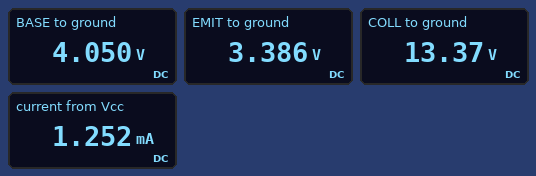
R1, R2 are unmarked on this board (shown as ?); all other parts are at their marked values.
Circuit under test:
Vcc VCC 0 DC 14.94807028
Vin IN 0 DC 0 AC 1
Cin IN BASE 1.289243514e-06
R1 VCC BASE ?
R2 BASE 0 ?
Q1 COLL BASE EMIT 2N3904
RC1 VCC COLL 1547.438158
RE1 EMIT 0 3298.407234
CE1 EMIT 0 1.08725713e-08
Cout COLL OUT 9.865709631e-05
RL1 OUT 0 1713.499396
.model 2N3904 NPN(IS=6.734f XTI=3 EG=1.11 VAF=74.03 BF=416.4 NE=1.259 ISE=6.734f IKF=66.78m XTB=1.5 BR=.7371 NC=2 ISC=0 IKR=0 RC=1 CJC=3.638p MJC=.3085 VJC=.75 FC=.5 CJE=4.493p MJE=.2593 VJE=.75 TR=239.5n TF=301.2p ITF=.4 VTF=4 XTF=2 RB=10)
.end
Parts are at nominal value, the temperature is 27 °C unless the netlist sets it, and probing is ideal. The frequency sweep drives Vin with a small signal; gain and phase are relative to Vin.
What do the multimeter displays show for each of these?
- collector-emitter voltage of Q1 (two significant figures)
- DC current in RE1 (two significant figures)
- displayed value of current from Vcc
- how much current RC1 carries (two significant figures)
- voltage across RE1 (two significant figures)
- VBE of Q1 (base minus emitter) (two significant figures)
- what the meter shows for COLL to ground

10 V
1.0 mA
1.252 mA
1.0 mA
3.4 V
660 mV
13.37 V
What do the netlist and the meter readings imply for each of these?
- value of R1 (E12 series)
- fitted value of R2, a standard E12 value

47 kΩ
18 kΩ
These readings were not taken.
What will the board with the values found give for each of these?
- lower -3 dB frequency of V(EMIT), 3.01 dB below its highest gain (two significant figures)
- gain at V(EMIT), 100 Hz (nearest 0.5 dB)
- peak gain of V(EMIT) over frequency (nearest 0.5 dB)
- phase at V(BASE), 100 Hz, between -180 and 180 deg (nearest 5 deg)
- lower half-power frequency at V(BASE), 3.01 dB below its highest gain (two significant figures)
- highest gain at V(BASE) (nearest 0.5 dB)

9.7 Hz
0 dB
0 dB
5 deg
9.7 Hz
0 dB
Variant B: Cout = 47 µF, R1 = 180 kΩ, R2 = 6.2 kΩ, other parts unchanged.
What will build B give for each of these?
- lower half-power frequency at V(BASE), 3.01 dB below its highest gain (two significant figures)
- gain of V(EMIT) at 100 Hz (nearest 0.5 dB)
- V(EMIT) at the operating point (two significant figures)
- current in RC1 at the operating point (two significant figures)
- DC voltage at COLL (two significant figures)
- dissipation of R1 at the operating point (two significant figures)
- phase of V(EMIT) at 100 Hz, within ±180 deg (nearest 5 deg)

21 Hz
-16.0 dB
5.0 mV
1.5 µA
15 V
1.2 mW
10 deg
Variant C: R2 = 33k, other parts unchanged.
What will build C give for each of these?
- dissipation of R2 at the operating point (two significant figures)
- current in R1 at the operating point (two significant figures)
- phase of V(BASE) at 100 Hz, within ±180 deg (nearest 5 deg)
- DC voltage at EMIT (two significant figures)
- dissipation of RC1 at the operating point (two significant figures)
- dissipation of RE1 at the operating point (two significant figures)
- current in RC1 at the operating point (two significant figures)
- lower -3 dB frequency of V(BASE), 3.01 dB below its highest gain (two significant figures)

1.1 mW
190 µA
5 deg
5.3 V
3.9 mW
8.5 mW
1.6 mA
6.6 Hz
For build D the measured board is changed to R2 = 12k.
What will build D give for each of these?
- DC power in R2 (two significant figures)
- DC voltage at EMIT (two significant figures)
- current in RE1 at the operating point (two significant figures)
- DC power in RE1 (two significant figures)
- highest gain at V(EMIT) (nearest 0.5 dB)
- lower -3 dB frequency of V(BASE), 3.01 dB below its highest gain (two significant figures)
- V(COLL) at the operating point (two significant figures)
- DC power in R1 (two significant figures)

750 µW
2.3 V
710 µA
1.7 mW
0 dB
13 Hz
14 V
3.0 mW
